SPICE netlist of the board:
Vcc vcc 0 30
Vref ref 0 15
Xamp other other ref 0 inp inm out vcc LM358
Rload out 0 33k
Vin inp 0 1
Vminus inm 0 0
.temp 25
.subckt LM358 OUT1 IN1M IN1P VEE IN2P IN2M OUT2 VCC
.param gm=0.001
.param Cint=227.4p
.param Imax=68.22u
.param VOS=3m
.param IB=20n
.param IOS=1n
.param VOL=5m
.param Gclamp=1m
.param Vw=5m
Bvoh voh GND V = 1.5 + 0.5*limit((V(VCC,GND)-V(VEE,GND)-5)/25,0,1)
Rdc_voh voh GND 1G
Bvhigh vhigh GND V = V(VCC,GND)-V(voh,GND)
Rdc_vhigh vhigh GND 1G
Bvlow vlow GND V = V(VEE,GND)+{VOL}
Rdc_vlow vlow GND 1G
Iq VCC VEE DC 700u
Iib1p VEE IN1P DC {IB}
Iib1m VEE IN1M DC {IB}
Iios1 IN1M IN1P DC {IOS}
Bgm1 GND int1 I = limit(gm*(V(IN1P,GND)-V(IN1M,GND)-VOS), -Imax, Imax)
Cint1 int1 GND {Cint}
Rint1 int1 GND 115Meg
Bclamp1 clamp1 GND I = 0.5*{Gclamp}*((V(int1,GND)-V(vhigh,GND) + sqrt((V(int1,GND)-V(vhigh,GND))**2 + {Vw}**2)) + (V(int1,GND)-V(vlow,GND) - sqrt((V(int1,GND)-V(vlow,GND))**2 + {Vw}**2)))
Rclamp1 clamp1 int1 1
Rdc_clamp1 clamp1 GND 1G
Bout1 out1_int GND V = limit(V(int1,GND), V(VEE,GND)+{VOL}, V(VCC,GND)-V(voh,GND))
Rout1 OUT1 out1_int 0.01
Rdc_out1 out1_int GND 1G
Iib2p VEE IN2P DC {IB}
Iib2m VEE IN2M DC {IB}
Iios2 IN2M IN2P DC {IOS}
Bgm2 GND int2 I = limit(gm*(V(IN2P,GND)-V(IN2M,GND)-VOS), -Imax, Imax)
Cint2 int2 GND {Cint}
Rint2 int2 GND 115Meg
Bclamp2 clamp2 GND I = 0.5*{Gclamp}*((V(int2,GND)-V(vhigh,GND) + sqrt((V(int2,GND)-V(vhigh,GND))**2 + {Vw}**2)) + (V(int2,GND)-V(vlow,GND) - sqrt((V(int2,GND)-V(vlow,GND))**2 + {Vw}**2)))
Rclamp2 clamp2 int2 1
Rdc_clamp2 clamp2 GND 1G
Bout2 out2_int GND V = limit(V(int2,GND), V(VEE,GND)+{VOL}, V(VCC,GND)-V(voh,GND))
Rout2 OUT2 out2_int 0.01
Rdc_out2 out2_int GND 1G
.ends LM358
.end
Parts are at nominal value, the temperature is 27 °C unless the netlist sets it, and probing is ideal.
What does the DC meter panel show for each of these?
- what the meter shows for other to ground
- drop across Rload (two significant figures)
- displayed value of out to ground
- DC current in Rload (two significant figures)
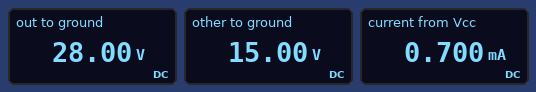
15.00 V
28 V
28.00 V
850 µA
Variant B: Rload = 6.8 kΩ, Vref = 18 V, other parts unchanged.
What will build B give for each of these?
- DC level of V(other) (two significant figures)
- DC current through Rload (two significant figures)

18 V
4.1 mA
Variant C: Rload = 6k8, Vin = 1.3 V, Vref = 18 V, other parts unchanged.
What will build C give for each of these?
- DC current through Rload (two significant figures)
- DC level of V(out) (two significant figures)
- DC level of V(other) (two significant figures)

4.1 mA
28 V
18 V
